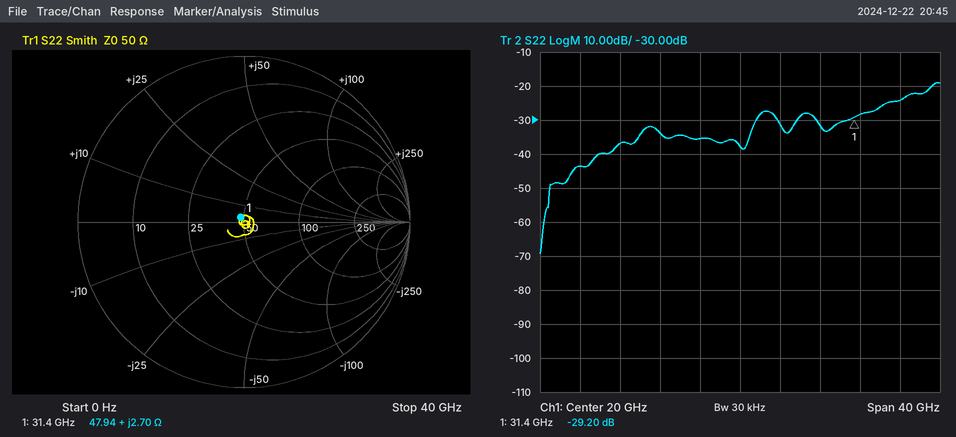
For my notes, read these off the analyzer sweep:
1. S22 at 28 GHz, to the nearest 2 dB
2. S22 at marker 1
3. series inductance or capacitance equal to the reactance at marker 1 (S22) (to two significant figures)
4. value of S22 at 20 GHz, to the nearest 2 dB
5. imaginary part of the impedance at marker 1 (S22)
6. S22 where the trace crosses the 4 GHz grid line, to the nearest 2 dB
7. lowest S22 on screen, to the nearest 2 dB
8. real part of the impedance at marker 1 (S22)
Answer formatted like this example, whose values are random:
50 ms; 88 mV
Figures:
-32 dB; -29.20 dB; 14 pH; -38 dB; +2.70 Ω; -44 dB; -70 dB; 47.94 Ω
